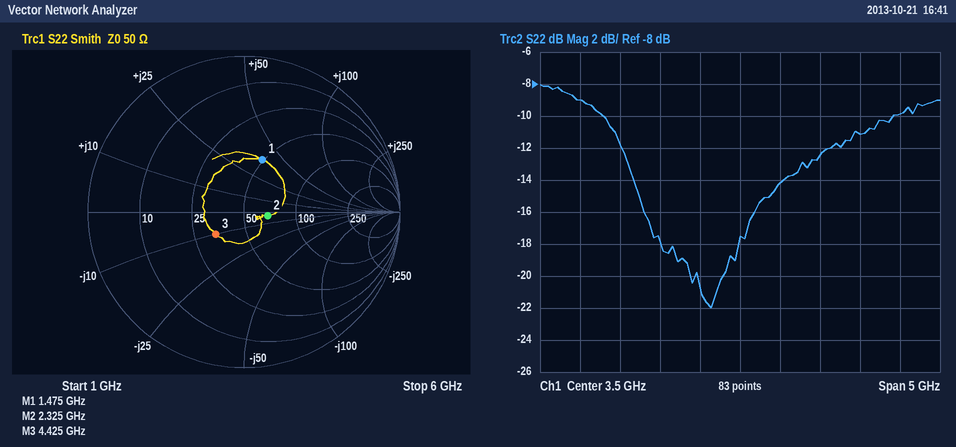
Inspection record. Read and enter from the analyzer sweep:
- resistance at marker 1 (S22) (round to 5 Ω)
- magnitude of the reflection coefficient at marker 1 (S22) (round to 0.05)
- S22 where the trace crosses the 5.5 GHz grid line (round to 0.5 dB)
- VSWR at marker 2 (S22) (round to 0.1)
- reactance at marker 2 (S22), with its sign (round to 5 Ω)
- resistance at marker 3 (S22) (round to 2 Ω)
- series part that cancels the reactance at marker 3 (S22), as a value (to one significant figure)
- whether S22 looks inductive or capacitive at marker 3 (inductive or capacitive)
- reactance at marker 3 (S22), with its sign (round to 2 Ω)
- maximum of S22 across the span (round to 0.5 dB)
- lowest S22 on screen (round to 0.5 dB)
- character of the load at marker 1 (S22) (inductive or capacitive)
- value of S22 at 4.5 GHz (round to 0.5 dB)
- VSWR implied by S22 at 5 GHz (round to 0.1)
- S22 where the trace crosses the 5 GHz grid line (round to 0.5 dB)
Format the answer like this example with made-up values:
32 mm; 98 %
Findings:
50 Ω; 0.35; -10.0 dB; 1.4; -5 Ω; 34 Ω; 400 pH; capacitive; -10 Ω; -8.0 dB; -22.0 dB; inductive; -12.5 dB; 1.8; -11.0 dB
